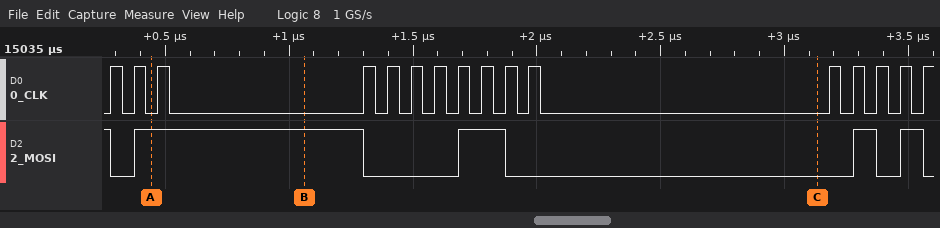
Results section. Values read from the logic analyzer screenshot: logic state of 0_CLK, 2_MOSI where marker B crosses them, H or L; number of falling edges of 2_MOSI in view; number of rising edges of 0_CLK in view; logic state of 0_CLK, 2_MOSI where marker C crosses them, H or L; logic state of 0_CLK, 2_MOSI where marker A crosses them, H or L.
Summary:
0_CLK=L, 2_MOSI=H
5
16
0_CLK=L, 2_MOSI=L
0_CLK=L, 2_MOSI=H
